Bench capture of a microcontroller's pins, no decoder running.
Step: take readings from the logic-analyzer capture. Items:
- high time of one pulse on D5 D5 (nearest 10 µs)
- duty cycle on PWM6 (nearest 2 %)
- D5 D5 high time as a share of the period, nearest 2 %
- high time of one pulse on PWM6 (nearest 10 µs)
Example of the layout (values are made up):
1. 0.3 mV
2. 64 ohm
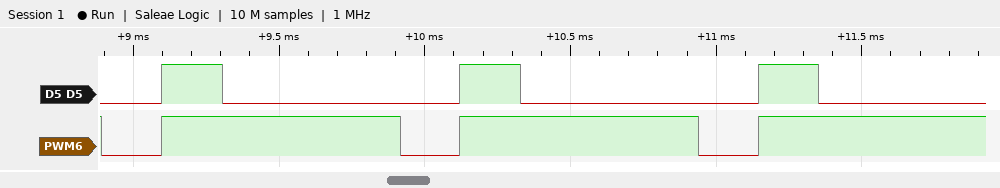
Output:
1. 210 µs
2. 80 %
3. 20 %
4. 820 µs
